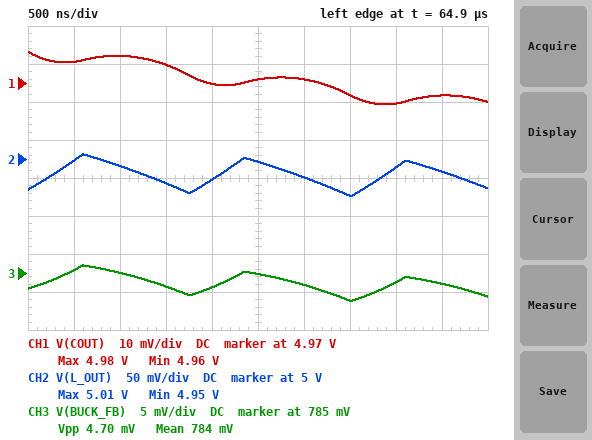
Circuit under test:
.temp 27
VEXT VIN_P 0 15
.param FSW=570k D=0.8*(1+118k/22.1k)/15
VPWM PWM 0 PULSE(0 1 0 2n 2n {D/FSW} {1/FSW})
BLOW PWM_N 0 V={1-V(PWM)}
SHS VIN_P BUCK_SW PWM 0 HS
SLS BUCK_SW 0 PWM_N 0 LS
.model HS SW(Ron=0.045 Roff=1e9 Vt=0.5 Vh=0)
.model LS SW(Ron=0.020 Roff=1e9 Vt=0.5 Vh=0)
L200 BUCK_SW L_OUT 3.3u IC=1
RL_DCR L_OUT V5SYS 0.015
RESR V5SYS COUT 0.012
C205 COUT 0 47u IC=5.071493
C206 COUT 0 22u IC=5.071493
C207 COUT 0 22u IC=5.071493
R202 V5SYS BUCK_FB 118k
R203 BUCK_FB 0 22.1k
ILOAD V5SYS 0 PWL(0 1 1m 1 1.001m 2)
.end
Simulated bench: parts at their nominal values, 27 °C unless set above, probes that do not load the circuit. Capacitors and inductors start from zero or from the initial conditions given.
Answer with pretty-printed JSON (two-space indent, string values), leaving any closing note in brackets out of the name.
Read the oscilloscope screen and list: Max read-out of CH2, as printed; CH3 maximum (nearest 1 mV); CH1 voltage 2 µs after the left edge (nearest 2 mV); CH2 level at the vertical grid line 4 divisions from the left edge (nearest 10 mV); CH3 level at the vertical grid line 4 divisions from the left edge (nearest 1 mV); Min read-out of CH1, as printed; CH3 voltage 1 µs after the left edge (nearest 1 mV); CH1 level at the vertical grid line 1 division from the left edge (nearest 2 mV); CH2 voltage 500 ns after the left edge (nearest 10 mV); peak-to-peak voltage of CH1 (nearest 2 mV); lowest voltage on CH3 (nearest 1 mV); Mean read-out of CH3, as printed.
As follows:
{
  "Max read-out of CH2, as printed": "5.01 V",
  "CH3 maximum": "786 mV",
  "CH1 voltage 2 µs after the left edge": "4.970 V",
  "CH2 level at the vertical grid line 4 divisions from the left edge": "4.97 V",
  "CH3 level at the vertical grid line 4 divisions from the left edge": "783 mV",
  "Min read-out of CH1, as printed": "4.96 V",
  "CH3 voltage 1 µs after the left edge": "785 mV",
  "CH1 level at the vertical grid line 1 division from the left edge": "4.976 V",
  "CH2 voltage 500 ns after the left edge": "5.00 V",
  "peak-to-peak voltage of CH1": "14 mV",
  "lowest voltage on CH3": "781 mV",
  "Mean read-out of CH3, as printed": "784 mV"
}
